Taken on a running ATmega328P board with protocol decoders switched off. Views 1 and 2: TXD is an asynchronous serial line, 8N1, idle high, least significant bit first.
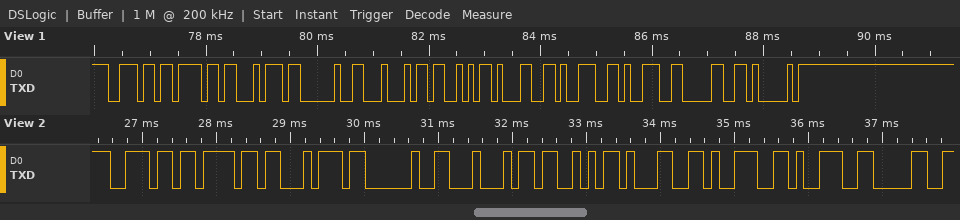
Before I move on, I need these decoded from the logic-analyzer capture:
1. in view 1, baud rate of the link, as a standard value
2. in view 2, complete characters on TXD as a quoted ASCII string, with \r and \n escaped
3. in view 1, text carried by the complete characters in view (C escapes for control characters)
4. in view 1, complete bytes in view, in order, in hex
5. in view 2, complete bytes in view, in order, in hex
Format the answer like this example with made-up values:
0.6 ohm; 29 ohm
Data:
9600 baud; "not DS1990"; "not DS1990A"; 6E 6F 74 20 44 53 31 39 39 30 41; 6E 6F 74 20 44 53 31 39 39 30
